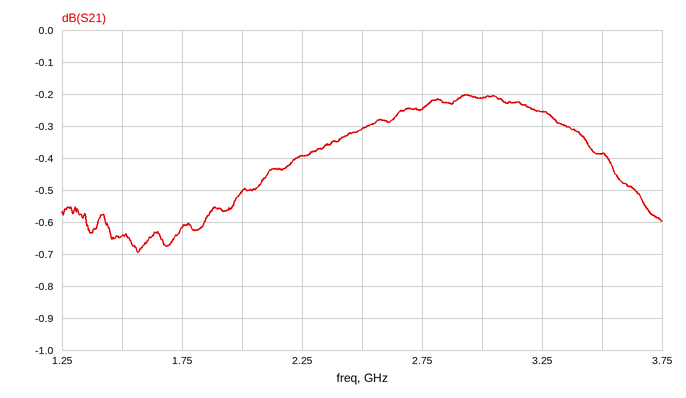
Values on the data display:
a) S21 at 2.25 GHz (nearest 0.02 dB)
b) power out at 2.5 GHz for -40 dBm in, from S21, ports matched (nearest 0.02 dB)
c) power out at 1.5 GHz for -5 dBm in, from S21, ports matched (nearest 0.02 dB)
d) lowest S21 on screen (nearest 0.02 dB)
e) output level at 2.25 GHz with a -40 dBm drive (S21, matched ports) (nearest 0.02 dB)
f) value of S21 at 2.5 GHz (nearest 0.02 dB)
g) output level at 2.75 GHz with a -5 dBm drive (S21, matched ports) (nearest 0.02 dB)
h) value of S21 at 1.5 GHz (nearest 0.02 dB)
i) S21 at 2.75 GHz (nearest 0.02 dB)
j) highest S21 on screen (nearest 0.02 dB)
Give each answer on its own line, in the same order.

-0.40 dB
-40.30 dBm
-5.64 dBm
-0.70 dB
-40.40 dBm
-0.30 dB
-5.24 dBm
-0.64 dB
-0.24 dB
-0.20 dB
